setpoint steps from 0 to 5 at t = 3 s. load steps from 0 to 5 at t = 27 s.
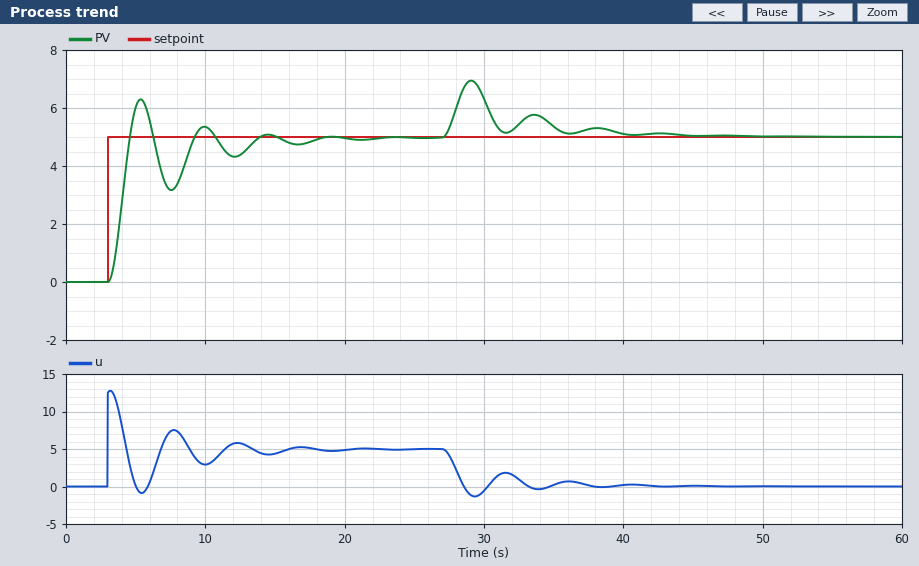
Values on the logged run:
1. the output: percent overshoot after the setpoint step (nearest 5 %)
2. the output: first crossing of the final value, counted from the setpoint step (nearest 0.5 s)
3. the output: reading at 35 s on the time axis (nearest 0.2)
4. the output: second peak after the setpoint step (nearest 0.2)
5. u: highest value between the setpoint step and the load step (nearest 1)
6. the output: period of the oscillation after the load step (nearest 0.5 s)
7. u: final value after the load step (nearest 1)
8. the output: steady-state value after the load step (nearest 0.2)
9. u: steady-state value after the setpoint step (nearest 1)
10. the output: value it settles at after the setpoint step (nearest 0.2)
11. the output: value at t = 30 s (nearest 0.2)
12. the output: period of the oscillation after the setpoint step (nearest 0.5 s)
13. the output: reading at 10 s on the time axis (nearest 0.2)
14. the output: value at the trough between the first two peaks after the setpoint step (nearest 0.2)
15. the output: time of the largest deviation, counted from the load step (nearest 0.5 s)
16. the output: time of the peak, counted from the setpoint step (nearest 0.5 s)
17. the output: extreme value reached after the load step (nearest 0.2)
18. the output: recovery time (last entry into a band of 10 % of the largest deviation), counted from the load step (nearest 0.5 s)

25 %
1.5 s
5.4
5.4
13
4.5 s
0
5.0
5
5.0
6.4
4.5 s
5.4
3.2
2.0 s
2.5 s
7.0
12.5 s
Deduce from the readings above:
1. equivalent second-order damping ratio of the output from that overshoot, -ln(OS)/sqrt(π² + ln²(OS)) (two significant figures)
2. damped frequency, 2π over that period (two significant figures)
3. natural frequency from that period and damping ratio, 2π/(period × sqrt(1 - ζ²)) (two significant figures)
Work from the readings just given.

0.40
1.4 rad/s
1.5 rad/s
